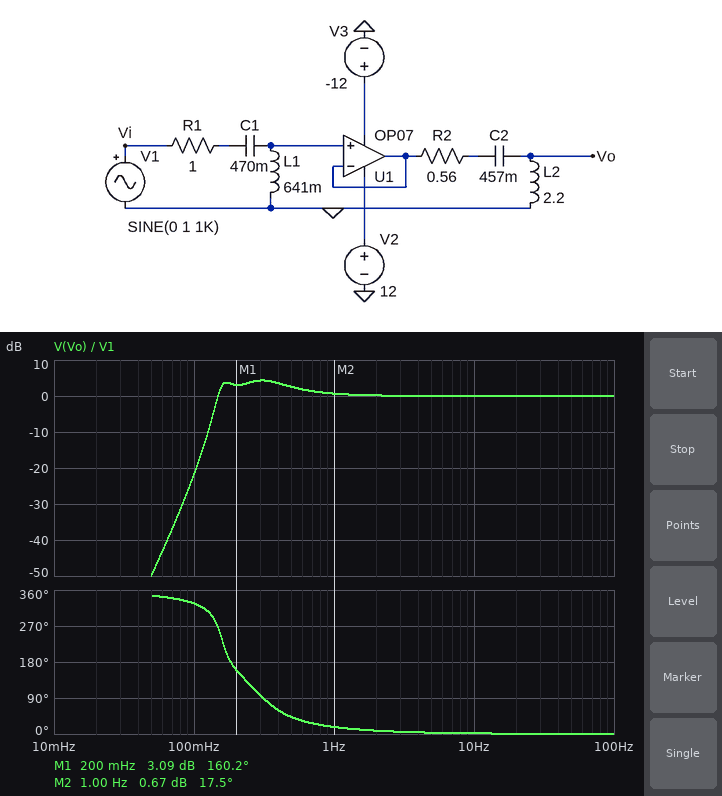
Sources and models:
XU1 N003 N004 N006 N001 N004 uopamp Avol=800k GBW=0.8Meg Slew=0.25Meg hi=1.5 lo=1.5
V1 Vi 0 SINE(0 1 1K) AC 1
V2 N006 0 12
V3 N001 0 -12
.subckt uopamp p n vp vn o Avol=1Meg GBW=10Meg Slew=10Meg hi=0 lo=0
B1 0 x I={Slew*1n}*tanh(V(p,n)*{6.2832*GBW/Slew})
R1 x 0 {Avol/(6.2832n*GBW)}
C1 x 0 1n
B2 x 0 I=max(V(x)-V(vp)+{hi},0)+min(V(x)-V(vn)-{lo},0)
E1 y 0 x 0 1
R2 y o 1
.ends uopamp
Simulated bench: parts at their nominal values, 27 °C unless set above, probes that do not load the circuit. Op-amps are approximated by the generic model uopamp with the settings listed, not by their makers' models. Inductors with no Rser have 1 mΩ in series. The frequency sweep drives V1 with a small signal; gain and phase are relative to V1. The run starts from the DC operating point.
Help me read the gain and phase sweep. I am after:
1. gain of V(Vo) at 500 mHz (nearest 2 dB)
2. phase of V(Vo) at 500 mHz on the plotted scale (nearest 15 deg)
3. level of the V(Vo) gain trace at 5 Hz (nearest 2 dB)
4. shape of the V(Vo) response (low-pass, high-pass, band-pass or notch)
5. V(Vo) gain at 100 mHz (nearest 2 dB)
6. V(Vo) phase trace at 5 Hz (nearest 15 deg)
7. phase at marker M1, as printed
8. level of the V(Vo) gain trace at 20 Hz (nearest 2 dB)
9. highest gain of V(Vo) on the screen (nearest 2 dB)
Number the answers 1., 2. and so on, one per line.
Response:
1. 2 dB
2. 45 deg
3. 0 dB
4. high-pass
5. -22 dB
6. 0 deg
7. 160.2 deg
8. 0 dB
9. 4 dB
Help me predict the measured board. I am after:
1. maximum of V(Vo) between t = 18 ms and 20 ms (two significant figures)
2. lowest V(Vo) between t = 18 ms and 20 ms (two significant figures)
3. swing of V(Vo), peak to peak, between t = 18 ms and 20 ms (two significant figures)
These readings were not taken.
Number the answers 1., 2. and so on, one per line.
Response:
1. 1.0 V
2. -1.0 V
3. 2.0 V
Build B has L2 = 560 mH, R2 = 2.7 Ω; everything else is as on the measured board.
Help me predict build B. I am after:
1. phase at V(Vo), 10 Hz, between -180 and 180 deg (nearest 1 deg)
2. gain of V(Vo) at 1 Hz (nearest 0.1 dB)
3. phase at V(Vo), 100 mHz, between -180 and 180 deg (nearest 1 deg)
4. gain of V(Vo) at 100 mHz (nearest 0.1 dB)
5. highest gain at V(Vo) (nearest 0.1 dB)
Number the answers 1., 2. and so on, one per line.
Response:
1. 6 deg
2. -1.0 dB
3. -60 deg
4. -39.3 dB
5. 0 dB
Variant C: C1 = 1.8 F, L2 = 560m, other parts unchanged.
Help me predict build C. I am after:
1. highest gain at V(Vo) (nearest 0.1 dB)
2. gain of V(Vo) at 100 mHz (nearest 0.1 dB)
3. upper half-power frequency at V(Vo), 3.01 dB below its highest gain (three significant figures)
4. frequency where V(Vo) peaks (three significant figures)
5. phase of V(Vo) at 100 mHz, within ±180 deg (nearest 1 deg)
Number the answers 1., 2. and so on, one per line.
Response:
1. 5.4 dB
2. -27.9 dB
3. 551 mHz
4. 342 mHz
5. -75 deg
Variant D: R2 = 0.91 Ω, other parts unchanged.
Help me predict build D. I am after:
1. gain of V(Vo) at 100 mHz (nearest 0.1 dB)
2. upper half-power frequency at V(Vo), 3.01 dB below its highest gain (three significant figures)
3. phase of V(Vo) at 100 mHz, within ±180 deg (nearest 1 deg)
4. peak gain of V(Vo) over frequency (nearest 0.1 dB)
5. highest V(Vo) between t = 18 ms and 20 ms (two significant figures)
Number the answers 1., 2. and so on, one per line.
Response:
1. -22.2 dB
2. 767 mHz
3. -42 deg
4. 4.1 dB
5. 1.0 V
